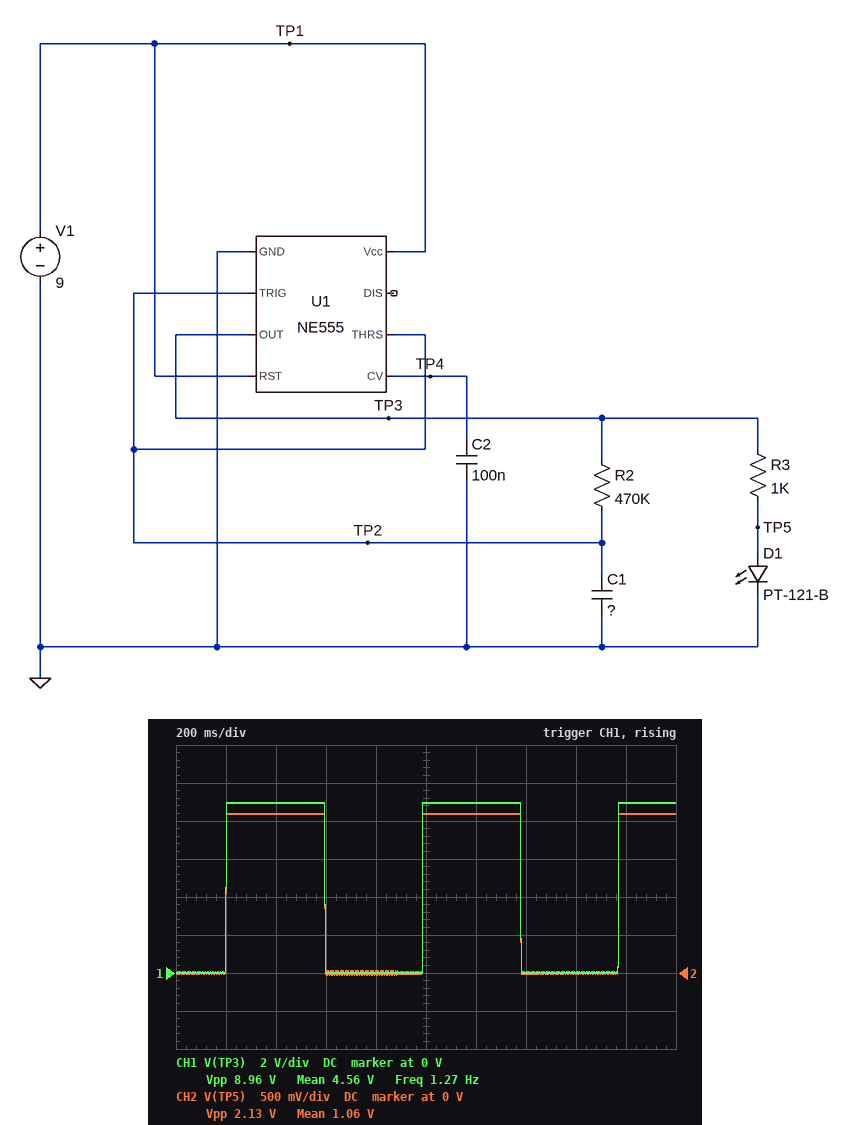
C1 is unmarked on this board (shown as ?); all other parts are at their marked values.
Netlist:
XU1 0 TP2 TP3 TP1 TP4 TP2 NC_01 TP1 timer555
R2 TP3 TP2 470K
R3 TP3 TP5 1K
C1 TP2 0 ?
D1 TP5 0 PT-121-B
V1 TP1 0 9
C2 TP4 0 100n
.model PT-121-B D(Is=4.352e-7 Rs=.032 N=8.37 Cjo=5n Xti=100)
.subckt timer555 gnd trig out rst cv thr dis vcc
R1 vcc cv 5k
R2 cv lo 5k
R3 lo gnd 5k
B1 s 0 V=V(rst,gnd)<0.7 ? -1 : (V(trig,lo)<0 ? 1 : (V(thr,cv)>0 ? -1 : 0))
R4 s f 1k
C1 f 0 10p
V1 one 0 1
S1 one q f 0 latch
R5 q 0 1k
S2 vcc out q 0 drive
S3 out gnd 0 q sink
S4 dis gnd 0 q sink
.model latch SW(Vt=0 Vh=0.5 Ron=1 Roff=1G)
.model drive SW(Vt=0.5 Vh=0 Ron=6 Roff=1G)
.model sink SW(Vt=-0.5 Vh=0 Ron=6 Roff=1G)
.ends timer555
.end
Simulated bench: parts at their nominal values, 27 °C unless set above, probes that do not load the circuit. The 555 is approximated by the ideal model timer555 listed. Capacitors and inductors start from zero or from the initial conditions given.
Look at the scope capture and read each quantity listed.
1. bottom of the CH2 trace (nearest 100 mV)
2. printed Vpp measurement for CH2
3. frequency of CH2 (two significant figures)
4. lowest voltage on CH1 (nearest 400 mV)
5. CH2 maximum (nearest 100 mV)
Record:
0 V
2.13 V
1.3 Hz
0 V
2.1 V
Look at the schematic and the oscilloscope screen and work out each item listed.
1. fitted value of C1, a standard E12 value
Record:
1.2 µF
